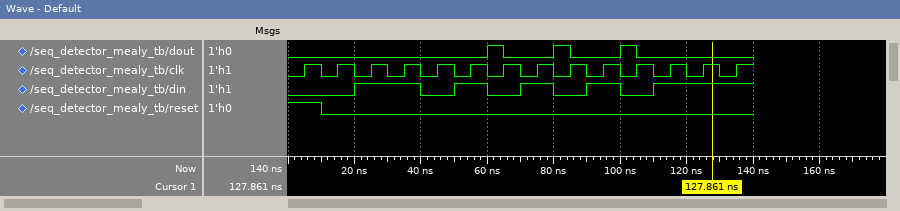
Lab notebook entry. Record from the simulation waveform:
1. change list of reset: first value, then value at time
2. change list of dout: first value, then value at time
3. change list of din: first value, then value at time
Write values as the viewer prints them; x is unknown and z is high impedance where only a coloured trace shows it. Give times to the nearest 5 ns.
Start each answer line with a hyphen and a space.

- 1, 0 at 10 ns
- 0, 1 at 60 ns, 0 at 65 ns, 1 at 80 ns, 0 at 85 ns, 1 at 100 ns, 0 at 105 ns
- 0, 1 at 20 ns, 0 at 40 ns, 1 at 50 ns, 0 at 60 ns, 1 at 70 ns, 0 at 80 ns, 1 at 90 ns, 0 at 100 ns, 1 at 110 ns
